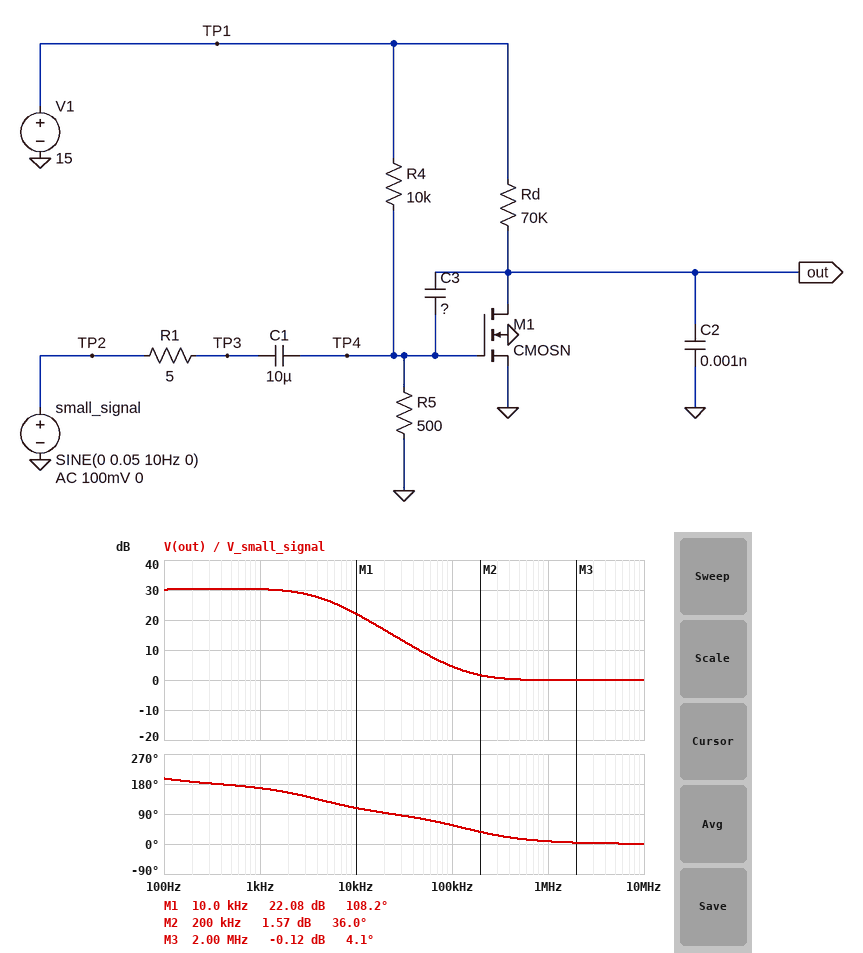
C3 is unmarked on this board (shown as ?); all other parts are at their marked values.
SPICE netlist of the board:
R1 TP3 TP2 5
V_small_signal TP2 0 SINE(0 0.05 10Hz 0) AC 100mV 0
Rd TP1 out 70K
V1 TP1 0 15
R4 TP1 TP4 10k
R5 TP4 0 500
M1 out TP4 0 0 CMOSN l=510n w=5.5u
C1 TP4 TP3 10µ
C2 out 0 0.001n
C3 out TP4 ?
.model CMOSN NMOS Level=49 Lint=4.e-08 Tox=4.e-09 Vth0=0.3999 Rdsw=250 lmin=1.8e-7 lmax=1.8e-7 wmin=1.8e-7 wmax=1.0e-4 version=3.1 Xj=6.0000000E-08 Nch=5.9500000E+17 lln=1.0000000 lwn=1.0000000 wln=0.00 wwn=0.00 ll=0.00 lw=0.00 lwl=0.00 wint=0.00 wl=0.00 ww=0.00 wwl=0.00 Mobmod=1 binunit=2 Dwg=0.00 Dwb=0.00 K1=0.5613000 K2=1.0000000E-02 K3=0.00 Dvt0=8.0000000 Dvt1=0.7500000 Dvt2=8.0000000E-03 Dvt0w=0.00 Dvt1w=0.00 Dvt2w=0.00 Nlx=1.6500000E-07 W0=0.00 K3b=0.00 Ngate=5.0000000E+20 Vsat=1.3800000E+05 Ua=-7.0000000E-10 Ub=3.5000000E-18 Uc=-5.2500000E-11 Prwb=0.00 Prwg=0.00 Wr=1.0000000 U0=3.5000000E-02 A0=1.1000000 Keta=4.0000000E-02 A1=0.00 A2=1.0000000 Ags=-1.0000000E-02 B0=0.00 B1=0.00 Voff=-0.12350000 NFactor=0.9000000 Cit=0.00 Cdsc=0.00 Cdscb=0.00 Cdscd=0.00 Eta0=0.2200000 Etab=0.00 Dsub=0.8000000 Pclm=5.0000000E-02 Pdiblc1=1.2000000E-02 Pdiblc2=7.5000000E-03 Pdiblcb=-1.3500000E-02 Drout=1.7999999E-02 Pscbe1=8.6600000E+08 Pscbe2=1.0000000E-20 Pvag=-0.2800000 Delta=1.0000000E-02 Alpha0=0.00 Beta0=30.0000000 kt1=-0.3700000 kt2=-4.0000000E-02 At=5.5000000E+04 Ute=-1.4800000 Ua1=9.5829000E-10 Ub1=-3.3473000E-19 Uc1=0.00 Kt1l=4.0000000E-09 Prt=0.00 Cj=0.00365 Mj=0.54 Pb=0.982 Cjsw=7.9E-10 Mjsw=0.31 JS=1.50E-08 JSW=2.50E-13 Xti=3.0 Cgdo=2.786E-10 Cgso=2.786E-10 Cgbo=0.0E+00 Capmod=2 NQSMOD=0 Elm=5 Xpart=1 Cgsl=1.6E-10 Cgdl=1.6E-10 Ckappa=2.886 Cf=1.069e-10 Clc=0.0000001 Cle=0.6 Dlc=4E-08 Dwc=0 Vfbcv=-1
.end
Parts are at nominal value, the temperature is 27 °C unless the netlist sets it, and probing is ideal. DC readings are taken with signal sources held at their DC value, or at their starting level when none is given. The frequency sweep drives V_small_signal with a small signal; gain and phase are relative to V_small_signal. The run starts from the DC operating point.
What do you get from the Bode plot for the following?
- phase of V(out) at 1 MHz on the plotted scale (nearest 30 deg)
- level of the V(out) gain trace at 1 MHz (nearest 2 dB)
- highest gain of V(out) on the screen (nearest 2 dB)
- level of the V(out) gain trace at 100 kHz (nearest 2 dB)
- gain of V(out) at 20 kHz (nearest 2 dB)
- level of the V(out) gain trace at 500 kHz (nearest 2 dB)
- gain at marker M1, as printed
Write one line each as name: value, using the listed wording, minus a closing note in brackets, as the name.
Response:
phase of V(out) at 1 MHz on the plotted scale: 0 deg
level of the V(out) gain trace at 1 MHz: 0 dB
highest gain of V(out) on the screen: 30 dB
level of the V(out) gain trace at 100 kHz: 4 dB
gain of V(out) at 20 kHz: 16 dB
level of the V(out) gain trace at 500 kHz: 0 dB
gain at marker M1, as printed: 22.08 dB
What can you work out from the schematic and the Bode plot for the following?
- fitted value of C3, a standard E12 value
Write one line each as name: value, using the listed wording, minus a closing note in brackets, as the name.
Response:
fitted value of C3, a standard E12 value: 1 nF
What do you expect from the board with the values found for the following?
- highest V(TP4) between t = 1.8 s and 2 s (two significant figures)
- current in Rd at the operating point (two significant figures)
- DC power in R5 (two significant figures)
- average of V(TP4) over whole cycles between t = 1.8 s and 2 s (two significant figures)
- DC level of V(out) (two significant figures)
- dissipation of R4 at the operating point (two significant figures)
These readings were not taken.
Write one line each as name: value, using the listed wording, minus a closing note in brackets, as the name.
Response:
highest V(TP4) between t = 1.8 s and 2 s: 730 mV
current in Rd at the operating point: 140 µA
DC power in R5: 1.0 mW
average of V(TP4) over whole cycles between t = 1.8 s and 2 s: 710 mV
DC level of V(out): 5.5 V
dissipation of R4 at the operating point: 20 mW
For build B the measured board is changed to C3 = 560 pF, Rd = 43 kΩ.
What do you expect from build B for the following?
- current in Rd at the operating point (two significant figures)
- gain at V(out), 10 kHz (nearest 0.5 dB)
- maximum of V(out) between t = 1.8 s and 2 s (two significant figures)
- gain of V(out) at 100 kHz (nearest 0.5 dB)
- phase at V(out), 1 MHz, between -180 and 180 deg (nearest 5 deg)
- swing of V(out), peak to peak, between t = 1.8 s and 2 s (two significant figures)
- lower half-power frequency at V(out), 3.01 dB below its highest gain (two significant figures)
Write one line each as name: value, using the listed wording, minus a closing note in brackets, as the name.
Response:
current in Rd at the operating point: 160 µA
gain at V(out), 10 kHz: 26.0 dB
maximum of V(out) between t = 1.8 s and 2 s: 8.4 V
gain of V(out) at 100 kHz: 9.5 dB
phase at V(out), 1 MHz, between -180 and 180 deg: 15 deg
swing of V(out), peak to peak, between t = 1.8 s and 2 s: 840 mV
lower half-power frequency at V(out), 3.01 dB below its highest gain: 33 Hz
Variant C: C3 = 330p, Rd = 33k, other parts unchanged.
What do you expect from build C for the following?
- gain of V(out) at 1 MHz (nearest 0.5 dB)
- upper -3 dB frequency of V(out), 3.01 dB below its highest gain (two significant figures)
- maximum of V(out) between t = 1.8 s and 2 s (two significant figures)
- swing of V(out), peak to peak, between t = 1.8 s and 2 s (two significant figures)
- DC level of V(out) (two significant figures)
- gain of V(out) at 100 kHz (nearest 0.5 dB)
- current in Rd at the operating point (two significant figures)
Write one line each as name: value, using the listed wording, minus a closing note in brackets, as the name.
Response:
gain of V(out) at 1 MHz: 1.0 dB
upper -3 dB frequency of V(out), 3.01 dB below its highest gain: 20 kHz
maximum of V(out) between t = 1.8 s and 2 s: 9.5 V
swing of V(out), peak to peak, between t = 1.8 s and 2 s: 750 mV
DC level of V(out): 9.2 V
gain of V(out) at 100 kHz: 14.0 dB
current in Rd at the operating point: 180 µA
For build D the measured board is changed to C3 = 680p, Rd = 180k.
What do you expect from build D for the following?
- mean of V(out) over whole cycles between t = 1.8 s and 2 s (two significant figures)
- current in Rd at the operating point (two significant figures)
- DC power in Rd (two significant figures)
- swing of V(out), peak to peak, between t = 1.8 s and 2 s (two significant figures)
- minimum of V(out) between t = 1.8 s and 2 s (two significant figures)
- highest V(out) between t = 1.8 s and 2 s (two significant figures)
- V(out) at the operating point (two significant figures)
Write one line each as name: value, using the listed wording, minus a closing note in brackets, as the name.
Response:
mean of V(out) over whole cycles between t = 1.8 s and 2 s: 610 mV
current in Rd at the operating point: 80 µA
DC power in Rd: 1.2 mW
swing of V(out), peak to peak, between t = 1.8 s and 2 s: 850 mV
minimum of V(out) between t = 1.8 s and 2 s: 230 mV
highest V(out) between t = 1.8 s and 2 s: 1.1 V
V(out) at the operating point: 570 mV
